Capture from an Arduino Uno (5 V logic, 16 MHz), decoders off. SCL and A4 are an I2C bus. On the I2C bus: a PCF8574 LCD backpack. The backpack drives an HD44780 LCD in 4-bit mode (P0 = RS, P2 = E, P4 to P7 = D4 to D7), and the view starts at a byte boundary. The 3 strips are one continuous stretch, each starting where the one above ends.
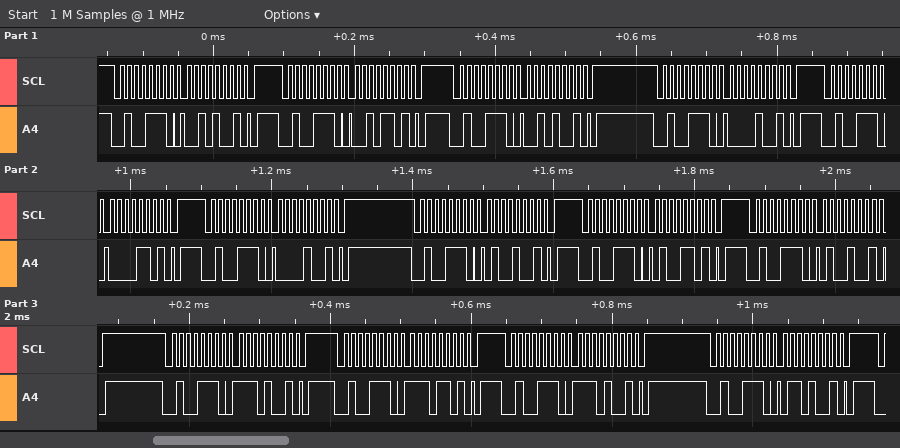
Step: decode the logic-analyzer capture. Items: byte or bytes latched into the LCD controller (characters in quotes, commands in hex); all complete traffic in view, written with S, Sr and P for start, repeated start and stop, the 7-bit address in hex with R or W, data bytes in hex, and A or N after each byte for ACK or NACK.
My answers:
' ' 'N'
S 27W A 29 A P S 27W A 2D A P S 27W A 29 A P S 27W A 09 A P S 27W A 0D A P S 27W A 09 A P S 27W A 49 A P S 27W A 4D A P S 27W A 49 A P S 27W A E9 A P S 27W A ED A P S 27W A E9 A P S 27W A 69 A P
